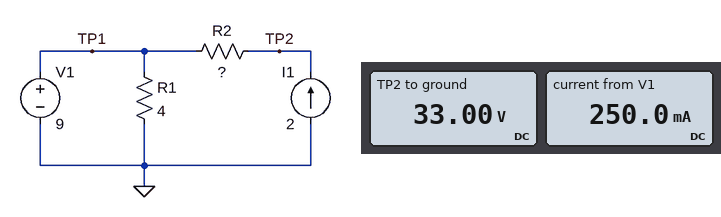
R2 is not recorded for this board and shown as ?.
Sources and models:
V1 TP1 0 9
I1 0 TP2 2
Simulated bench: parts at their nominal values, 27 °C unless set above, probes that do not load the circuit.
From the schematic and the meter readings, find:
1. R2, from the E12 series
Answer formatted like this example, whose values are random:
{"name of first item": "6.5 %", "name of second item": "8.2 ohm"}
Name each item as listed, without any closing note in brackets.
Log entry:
{"R2, from the E12 series": "12 Ω"}
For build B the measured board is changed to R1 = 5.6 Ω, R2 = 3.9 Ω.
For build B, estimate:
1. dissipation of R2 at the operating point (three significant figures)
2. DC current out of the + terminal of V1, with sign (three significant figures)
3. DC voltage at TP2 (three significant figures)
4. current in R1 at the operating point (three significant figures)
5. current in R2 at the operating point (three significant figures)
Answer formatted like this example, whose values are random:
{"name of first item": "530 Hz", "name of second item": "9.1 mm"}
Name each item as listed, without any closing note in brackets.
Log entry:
{"dissipation of R2 at the operating point": "15.6 W", "DC current out of the + terminal of V1, with sign": "-393 mA", "DC voltage at TP2": "16.8 V", "current in R1 at the operating point": "1.61 A", "current in R2 at the operating point": "2.00 A"}
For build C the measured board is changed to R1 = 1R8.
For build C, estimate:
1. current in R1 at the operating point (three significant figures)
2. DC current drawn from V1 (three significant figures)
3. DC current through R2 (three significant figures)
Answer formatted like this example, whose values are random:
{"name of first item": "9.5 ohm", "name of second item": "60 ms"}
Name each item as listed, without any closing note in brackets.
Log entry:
{"current in R1 at the operating point": "5.00 A", "DC current drawn from V1": "3.00 A", "DC current through R2": "2.00 A"}
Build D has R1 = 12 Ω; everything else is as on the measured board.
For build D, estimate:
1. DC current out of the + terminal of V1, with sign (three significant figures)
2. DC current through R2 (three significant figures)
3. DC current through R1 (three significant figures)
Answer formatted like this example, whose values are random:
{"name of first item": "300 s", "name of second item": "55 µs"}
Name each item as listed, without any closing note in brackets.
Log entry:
{"DC current out of the + terminal of V1, with sign": "-1.25 A", "DC current through R2": "2.00 A", "DC current through R1": "750 mA"}
